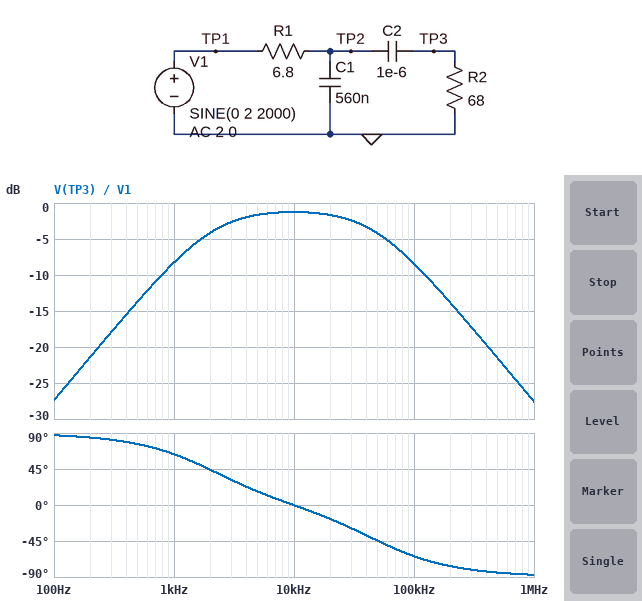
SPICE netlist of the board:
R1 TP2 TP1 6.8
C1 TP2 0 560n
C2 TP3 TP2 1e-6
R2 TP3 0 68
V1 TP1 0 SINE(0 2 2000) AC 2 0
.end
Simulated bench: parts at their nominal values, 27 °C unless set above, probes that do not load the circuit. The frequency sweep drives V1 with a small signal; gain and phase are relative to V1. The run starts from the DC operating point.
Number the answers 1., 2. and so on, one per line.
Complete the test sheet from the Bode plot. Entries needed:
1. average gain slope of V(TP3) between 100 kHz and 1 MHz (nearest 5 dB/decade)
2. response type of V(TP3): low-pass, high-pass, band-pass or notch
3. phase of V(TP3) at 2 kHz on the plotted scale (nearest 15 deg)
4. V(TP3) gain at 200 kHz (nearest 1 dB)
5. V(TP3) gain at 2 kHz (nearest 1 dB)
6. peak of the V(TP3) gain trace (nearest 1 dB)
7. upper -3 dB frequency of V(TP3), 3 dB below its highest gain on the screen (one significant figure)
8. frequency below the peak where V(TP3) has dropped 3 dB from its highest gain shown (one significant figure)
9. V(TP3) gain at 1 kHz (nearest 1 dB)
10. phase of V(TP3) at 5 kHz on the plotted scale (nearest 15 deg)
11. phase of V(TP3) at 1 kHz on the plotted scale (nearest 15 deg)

1. -20 dB/decade
2. band-pass
3. 45 deg
4. -14 dB
5. -4 dB
6. -1 dB
7. 50 kHz
8. 2 kHz
9. -8 dB
10. 15 deg
11. 60 deg
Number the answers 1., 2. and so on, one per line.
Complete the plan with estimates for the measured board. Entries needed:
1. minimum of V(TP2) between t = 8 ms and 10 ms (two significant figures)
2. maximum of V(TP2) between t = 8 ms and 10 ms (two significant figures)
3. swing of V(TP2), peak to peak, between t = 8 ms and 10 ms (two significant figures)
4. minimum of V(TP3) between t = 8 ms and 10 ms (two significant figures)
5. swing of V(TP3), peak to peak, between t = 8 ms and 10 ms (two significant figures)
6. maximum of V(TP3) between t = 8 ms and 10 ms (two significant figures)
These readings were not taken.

1. -1.9 V
2. 1.9 V
3. 3.8 V
4. -1.2 V
5. 2.5 V
6. 1.2 V
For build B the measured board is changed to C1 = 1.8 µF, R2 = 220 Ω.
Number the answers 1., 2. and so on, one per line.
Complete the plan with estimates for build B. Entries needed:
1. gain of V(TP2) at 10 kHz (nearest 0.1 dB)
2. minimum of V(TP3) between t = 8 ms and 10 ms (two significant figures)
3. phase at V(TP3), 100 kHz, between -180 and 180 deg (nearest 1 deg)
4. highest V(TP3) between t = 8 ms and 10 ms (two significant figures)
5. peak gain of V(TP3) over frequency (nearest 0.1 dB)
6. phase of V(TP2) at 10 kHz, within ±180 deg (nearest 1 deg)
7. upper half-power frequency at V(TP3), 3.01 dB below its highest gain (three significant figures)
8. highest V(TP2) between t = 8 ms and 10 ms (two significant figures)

1. -2.2 dB
2. -1.8 V
3. -82 deg
4. 1.8 V
5. -0.7 dB
6. -37 deg
7. 14.8 kHz
8. 1.9 V
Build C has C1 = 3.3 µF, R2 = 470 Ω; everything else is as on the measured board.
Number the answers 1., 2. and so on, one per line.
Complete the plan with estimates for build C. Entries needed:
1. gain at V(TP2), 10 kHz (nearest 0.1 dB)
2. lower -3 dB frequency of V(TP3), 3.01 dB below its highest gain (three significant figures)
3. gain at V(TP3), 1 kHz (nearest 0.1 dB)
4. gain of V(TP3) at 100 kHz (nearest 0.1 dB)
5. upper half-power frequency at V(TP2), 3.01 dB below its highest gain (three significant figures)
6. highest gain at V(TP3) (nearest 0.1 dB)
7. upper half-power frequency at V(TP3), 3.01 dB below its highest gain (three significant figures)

1. -4.8 dB
2. 306 Hz
3. -0.7 dB
4. -23.0 dB
5. 6.98 kHz
6. -0.5 dB
7. 7.84 kHz
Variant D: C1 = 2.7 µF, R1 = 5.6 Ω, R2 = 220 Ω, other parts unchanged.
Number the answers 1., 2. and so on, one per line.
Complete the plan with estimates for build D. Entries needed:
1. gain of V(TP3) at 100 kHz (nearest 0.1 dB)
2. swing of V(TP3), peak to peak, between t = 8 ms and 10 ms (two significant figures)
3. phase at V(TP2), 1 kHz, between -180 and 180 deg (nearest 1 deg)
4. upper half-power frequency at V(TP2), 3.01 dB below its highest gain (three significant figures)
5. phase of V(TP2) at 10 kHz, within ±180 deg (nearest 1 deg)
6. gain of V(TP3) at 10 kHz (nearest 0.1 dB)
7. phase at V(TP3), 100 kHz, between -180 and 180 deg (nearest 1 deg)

1. -19.6 dB
2. 3.6 V
3. -6 deg
4. 10.2 kHz
5. -43 deg
6. -2.9 dB
7. -83 deg
